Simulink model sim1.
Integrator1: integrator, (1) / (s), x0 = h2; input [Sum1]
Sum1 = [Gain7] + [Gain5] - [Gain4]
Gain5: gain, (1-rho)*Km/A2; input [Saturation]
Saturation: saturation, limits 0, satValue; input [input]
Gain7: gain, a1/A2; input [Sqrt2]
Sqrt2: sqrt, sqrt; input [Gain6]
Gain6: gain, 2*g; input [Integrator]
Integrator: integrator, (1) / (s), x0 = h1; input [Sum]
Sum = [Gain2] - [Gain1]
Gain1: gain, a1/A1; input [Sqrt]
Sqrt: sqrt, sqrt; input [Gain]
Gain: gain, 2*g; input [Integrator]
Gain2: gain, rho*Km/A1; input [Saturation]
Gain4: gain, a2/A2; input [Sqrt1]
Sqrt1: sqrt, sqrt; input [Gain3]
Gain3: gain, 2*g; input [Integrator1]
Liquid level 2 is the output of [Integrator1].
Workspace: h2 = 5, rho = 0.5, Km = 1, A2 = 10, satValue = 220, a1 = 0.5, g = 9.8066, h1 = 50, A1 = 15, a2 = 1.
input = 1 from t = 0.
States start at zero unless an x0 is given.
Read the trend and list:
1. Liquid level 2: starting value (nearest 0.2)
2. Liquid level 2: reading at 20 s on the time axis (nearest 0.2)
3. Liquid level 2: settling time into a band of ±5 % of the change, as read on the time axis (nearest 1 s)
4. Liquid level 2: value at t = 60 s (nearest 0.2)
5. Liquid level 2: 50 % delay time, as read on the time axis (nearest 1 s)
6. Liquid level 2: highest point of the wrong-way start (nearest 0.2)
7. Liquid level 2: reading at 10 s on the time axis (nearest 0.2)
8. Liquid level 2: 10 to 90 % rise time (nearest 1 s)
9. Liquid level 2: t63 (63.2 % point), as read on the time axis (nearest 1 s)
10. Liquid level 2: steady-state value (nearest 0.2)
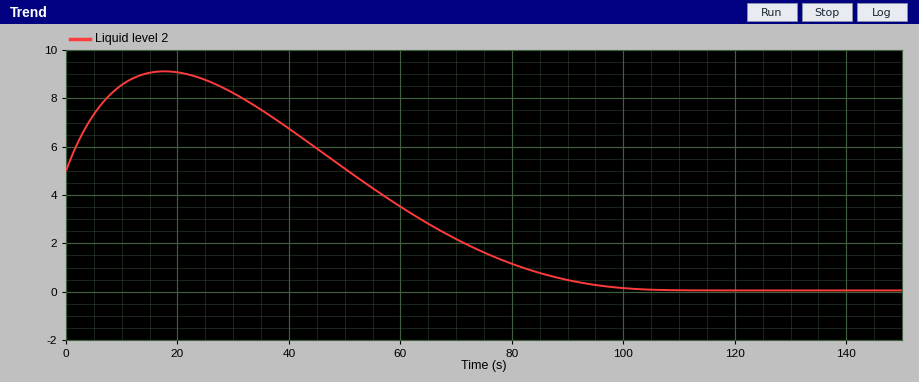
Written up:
5.0
9.0
94 s
3.6
67 s
9.2
8.6
35 s
73 s
0.0
